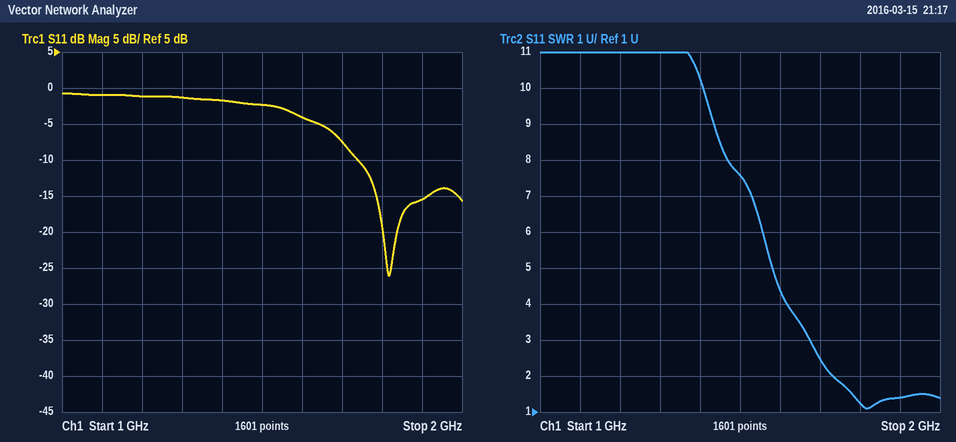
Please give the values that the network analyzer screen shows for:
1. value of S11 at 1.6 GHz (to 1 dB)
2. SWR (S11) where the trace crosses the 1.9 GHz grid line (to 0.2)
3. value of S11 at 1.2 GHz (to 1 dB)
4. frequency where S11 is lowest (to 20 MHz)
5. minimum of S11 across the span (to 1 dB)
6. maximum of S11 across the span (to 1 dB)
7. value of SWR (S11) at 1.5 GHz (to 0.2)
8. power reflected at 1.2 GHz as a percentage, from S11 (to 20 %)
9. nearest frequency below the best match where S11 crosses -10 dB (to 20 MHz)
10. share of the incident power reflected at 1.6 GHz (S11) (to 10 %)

-4 dB
1.4
-1 dB
1.82 GHz
-26 dB
-1 dB
7.6
80 %
1.74 GHz
40 %
